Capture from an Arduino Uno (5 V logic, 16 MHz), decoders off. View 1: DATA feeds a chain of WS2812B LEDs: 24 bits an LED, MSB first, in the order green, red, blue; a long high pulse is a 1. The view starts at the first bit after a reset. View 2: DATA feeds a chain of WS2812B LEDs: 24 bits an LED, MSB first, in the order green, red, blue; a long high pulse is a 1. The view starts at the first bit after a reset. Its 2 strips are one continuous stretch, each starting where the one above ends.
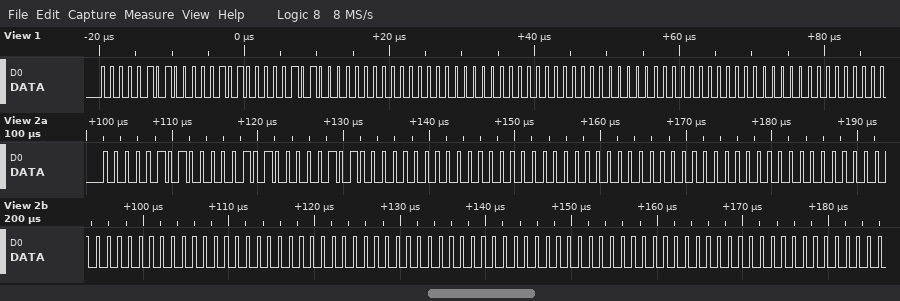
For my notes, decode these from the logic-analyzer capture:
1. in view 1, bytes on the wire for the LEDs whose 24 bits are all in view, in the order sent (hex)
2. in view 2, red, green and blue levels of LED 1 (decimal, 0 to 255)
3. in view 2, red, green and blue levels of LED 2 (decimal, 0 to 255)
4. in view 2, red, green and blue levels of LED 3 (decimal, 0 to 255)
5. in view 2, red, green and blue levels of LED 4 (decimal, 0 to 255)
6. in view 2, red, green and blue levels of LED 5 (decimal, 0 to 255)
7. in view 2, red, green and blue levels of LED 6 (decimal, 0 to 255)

05 05 05 00 00 00 00 00 00
5, 5, 5
0, 0, 0
0, 0, 0
0, 0, 0
0, 0, 0
0, 0, 0
